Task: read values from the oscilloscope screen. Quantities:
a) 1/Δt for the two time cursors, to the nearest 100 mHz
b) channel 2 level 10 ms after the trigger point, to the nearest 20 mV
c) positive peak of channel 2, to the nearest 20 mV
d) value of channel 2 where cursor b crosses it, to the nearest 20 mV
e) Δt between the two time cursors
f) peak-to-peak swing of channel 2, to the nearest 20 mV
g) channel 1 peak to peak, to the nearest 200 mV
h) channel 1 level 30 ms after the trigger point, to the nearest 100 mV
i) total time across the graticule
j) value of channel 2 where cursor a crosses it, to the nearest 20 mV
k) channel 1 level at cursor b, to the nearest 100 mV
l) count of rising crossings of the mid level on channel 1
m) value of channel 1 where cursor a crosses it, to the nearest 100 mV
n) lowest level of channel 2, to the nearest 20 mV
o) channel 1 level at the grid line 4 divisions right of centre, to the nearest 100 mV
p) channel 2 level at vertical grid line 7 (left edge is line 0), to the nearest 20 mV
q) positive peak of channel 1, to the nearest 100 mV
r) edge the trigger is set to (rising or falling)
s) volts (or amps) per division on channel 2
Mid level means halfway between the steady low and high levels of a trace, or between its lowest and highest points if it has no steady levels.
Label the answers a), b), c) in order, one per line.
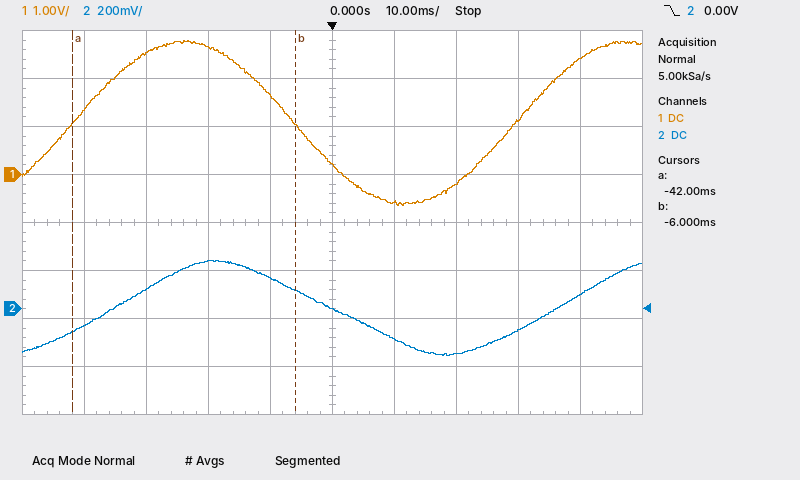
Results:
a) 27.8 Hz
b) -120 mV
c) 200 mV
d) 80 mV
e) 36 ms
f) 400 mV
g) 3.4 V
h) 1.1 V
i) 100 ms
j) -100 mV
k) 1.0 V
l) 2
m) 1.1 V
n) -200 mV
o) 2.4 V
p) -180 mV
q) 2.8 V
r) falling
s) 200 mV
